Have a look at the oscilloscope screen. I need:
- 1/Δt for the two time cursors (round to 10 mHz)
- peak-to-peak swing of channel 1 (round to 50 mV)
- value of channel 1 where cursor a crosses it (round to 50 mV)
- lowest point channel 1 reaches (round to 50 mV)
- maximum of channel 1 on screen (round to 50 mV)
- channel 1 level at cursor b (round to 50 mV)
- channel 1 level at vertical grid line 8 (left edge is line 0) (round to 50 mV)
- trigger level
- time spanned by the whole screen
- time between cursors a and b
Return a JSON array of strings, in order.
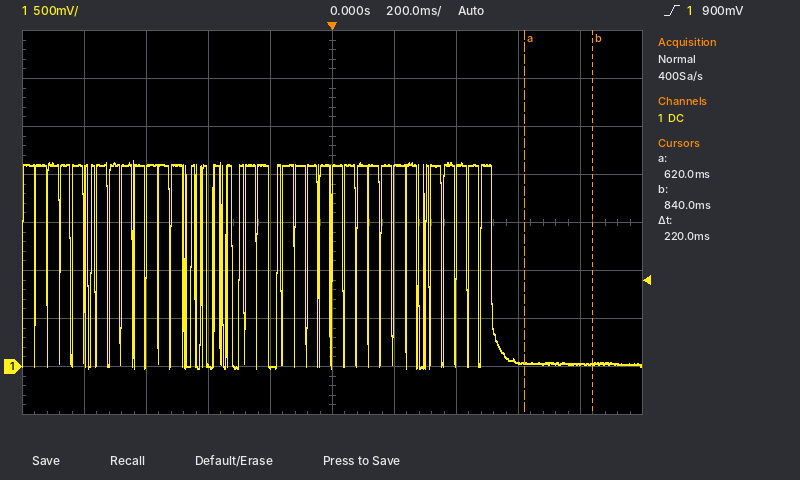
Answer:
["4.55 Hz", "2.15 V", "50 mV", "0 mV", "2.15 V", "50 mV", "50 mV", "900 mV", "2 s", "220 ms"]
